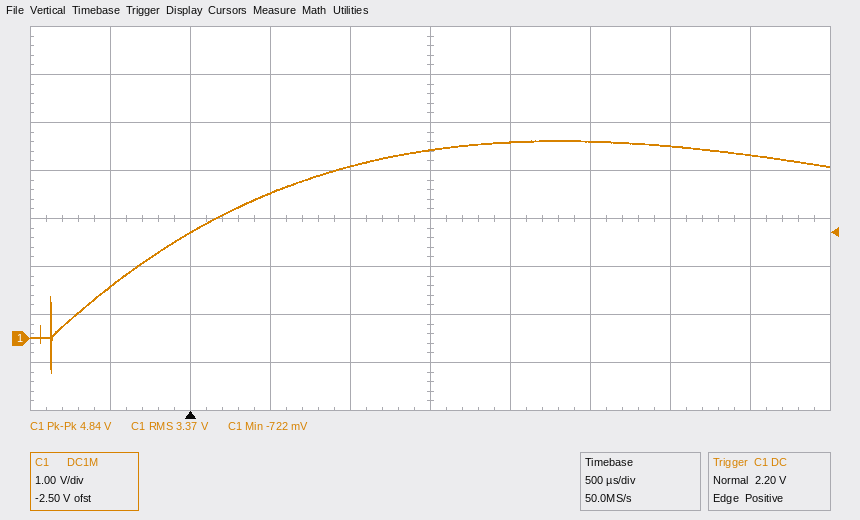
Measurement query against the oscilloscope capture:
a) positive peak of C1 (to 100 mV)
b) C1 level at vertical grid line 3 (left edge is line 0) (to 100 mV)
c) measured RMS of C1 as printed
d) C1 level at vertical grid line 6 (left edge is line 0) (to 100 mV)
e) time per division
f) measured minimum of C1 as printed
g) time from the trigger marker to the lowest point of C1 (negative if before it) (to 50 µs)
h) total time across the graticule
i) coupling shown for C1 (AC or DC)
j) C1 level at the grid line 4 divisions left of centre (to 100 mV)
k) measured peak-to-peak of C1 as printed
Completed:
4.1 V
3.0 V
3.37 V
4.1 V
500 µs
-722 mV
-850 µs
5 ms
DC
1.1 V
4.84 V
